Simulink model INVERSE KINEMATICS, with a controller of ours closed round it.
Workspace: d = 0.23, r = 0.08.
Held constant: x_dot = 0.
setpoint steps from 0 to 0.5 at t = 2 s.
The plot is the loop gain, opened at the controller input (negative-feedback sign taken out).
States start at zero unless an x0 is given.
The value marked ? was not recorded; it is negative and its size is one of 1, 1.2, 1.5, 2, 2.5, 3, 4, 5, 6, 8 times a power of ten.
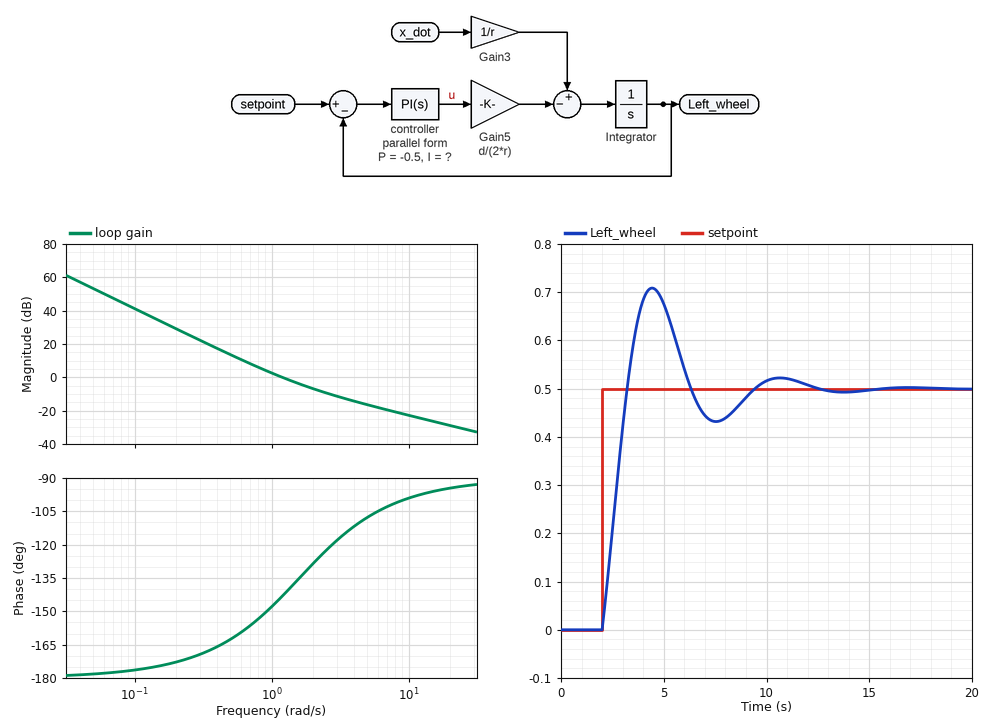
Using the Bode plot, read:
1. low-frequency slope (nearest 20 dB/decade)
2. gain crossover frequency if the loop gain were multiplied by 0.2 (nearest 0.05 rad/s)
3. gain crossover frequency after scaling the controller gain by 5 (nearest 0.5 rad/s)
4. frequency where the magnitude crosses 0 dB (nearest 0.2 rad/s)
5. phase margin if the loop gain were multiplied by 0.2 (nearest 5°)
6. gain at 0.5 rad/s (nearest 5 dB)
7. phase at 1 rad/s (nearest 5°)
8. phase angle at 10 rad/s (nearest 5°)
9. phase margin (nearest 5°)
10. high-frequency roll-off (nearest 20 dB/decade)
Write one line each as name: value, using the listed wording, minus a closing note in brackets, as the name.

low-frequency slope: -40 dB/decade
gain crossover frequency if the loop gain were multiplied by 0.2: 0.50 rad/s
gain crossover frequency after scaling the controller gain by 5: 4.0 rad/s
frequency where the magnitude crosses 0 dB: 1.2 rad/s
phase margin if the loop gain were multiplied by 0.2: 15°
gain at 0.5 rad/s: 15 dB
phase at 1 rad/s: -150°
phase angle at 10 rad/s: -100°
phase margin: 35°
high-frequency roll-off: -20 dB/decade
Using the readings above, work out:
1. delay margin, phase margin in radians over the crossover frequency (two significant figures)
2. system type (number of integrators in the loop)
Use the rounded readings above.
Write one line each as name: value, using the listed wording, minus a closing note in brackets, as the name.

delay margin, phase margin in radians over the crossover frequency: 0.51 s
system type: 2
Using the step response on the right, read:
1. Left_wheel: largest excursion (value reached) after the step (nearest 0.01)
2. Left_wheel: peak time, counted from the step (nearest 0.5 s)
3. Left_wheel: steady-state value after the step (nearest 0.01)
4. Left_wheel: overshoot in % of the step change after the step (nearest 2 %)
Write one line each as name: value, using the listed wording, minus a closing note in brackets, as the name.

Left_wheel: largest excursion (value reached) after the step: 0.71
Left_wheel: peak time, counted from the step: 2.5 s
Left_wheel: steady-state value after the step: 0.50
Left_wheel: overshoot in % of the step change after the step: 42 %
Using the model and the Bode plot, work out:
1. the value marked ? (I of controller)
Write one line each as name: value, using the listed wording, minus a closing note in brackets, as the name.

the value marked ?: -0.8
